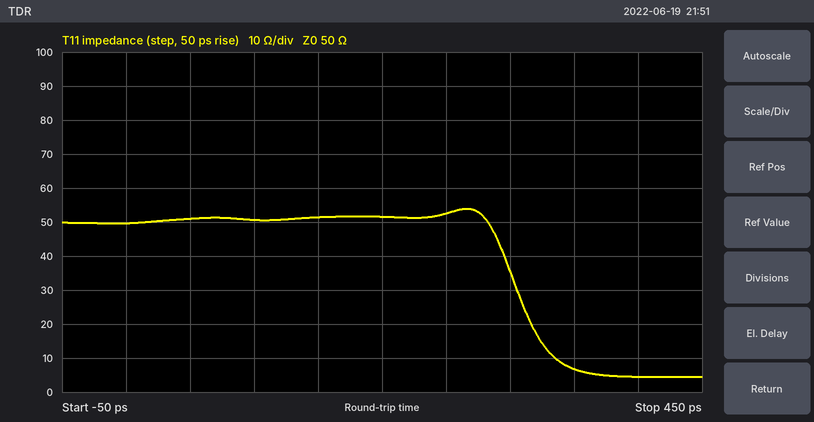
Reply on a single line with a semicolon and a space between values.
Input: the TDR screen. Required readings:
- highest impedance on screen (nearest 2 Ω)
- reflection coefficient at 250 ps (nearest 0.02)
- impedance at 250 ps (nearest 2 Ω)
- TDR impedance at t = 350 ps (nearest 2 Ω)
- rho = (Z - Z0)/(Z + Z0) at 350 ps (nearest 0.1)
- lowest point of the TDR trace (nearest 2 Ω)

54 Ω; +0.02; 52 Ω; 6 Ω; -0.8; 4 Ω
